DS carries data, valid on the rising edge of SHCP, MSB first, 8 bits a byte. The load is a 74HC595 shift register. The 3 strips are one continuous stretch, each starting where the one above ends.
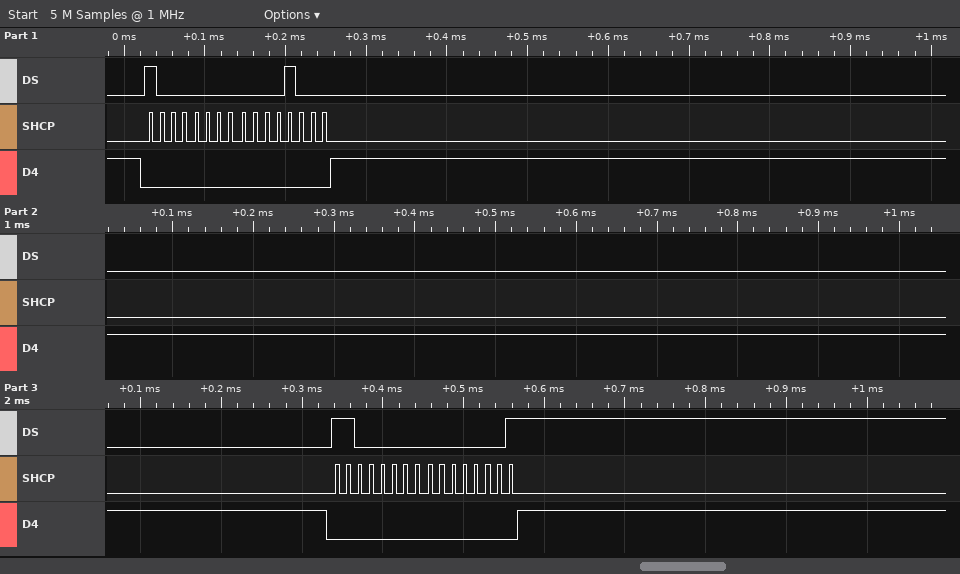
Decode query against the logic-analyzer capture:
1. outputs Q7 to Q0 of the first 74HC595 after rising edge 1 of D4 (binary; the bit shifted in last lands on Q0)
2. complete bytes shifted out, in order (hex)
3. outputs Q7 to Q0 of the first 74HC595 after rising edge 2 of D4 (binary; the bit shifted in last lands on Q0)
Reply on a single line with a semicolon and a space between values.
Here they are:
00001000; 80 08 C0 01; 00000001
